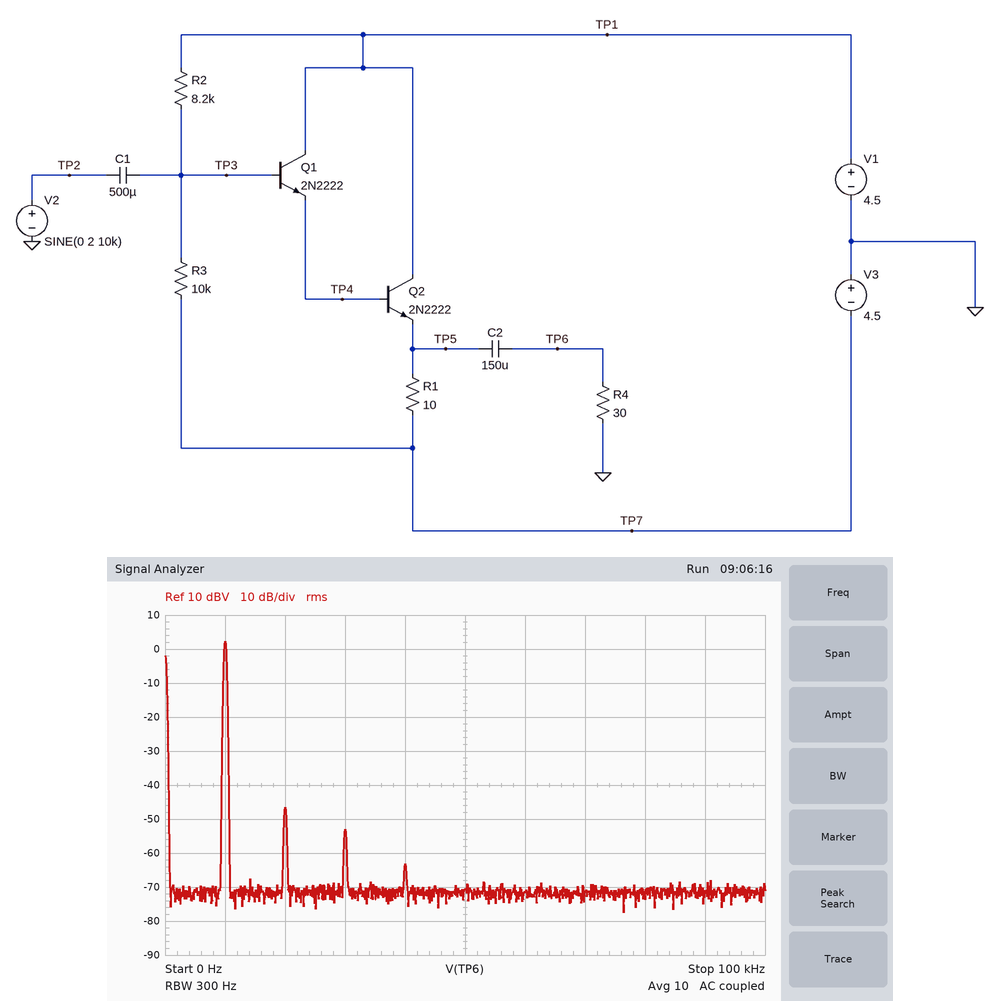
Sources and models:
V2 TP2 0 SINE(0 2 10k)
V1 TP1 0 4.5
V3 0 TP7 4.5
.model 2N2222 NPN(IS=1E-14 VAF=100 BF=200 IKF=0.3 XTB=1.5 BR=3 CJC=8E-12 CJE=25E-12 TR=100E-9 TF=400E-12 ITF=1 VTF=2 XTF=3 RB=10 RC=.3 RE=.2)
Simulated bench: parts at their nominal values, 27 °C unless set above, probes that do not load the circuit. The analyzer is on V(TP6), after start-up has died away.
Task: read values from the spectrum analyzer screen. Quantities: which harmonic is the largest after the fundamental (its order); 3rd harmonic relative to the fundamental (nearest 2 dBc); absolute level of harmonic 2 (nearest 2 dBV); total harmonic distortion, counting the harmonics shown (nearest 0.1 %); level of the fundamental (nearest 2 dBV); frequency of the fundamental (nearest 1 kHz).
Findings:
2
-56 dBc
-46 dBV
0.4 %
2 dBV
10 kHz
